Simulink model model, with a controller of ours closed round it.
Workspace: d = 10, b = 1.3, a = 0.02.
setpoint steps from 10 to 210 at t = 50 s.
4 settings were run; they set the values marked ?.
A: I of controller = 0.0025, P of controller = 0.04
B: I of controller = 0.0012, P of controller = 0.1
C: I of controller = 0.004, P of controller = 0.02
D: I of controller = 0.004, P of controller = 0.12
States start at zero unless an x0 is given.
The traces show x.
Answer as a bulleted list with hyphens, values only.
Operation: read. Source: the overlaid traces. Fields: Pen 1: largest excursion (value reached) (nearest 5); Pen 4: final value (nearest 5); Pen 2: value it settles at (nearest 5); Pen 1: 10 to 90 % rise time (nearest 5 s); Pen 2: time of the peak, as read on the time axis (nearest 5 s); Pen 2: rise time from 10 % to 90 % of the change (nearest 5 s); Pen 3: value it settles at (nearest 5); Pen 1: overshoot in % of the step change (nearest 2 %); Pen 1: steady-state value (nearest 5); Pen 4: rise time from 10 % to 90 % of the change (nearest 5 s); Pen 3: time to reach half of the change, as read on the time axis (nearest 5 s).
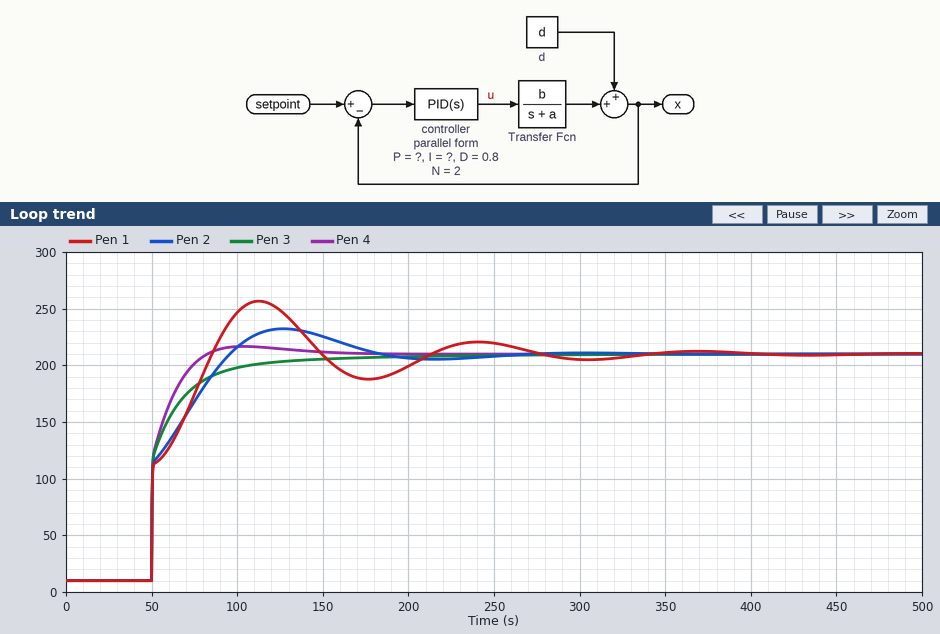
- 255
- 210
- 210
- 30 s
- 125 s
- 35 s
- 210
- 24 %
- 210
- 20 s
- 50 s
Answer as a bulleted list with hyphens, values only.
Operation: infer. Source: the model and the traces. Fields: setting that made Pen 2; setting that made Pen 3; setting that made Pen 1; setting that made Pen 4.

- A
- B
- C
- D
